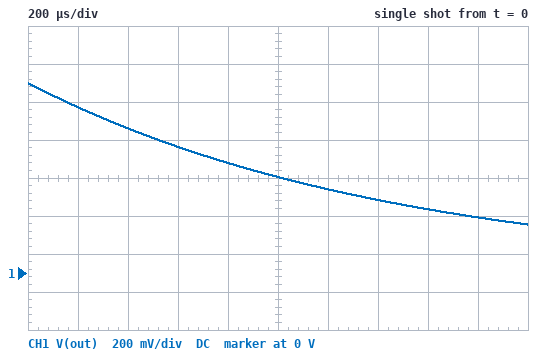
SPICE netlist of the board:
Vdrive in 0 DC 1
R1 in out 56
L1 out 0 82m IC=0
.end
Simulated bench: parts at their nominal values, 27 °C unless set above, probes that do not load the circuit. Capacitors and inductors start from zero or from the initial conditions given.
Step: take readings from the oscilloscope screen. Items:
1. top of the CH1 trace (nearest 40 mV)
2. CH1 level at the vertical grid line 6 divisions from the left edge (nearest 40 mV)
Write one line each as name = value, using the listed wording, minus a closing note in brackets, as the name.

top of the CH1 trace = 1.00 V
CH1 level at the vertical grid line 6 divisions from the left edge = 440 mV
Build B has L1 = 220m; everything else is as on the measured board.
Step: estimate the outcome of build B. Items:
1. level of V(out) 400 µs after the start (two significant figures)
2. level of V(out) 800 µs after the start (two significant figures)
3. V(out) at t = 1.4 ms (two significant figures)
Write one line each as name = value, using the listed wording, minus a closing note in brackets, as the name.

level of V(out) 400 µs after the start = 900 mV
level of V(out) 800 µs after the start = 820 mV
V(out) at t = 1.4 ms = 700 mV
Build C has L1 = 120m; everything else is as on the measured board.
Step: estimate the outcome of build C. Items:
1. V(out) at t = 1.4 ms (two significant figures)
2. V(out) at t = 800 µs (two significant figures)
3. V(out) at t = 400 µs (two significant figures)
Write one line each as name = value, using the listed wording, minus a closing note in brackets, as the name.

V(out) at t = 1.4 ms = 520 mV
V(out) at t = 800 µs = 690 mV
V(out) at t = 400 µs = 830 mV
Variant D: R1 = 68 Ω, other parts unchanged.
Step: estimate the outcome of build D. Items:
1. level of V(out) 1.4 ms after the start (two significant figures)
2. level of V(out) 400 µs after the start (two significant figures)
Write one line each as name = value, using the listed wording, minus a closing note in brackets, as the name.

level of V(out) 1.4 ms after the start = 310 mV
level of V(out) 400 µs after the start = 720 mV
